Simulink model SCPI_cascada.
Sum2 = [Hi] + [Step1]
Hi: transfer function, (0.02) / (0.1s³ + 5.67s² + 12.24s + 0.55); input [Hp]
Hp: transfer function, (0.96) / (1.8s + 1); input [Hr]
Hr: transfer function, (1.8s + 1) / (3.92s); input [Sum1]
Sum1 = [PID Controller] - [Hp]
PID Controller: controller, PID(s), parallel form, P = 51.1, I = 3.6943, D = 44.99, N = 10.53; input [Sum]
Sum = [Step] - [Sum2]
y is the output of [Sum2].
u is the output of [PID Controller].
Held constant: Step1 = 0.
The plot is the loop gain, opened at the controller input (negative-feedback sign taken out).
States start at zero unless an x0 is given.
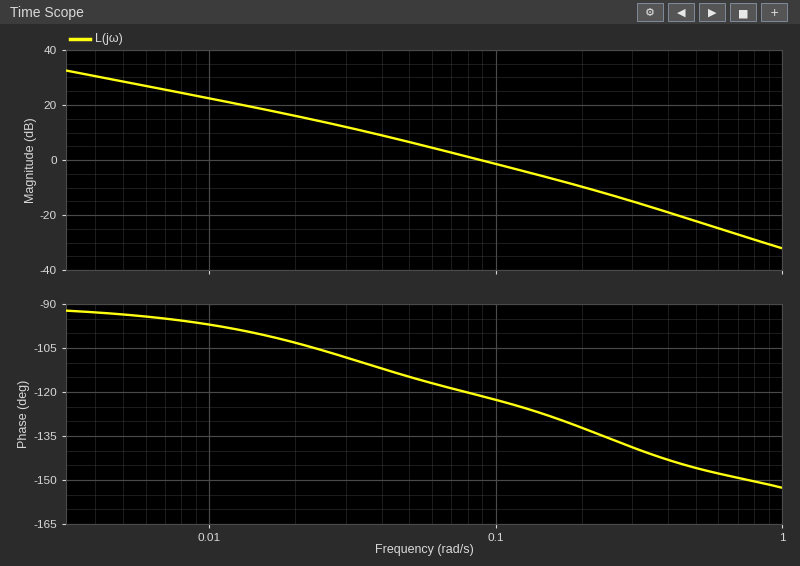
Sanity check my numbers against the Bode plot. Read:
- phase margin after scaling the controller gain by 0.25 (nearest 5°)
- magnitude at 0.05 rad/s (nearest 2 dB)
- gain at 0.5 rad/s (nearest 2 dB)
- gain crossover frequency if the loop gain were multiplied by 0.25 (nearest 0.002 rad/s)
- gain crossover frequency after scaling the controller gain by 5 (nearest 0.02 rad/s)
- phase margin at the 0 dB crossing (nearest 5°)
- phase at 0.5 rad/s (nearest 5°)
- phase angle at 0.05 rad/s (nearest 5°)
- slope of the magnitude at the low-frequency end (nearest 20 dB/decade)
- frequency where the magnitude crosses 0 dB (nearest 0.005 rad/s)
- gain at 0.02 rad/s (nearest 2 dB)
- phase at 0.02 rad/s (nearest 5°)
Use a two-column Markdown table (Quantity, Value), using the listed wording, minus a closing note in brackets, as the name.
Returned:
| Quantity | Value |
|---|---|
| phase margin after scaling the controller gain by 0.25 | 70° |
| magnitude at 0.05 rad/s | 6 dB |
| gain at 0.5 rad/s | -22 dB |
| gain crossover frequency if the loop gain were multiplied by 0.25 | 0.030 rad/s |
| gain crossover frequency after scaling the controller gain by 5 | 0.28 rad/s |
| phase margin at the 0 dB crossing | 60° |
| phase at 0.5 rad/s | -145° |
| phase angle at 0.05 rad/s | -115° |
| slope of the magnitude at the low-frequency end | -20 dB/decade |
| frequency where the magnitude crosses 0 dB | 0.090 rad/s |
| gain at 0.02 rad/s | 16 dB |
| phase at 0.02 rad/s | -105° |
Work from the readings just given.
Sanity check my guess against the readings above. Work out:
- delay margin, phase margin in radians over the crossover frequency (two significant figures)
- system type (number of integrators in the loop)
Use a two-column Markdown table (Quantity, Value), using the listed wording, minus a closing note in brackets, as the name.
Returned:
| Quantity | Value |
|---|---|
| delay margin, phase margin in radians over the crossover frequency | 12 s |
| system type | 1 |
